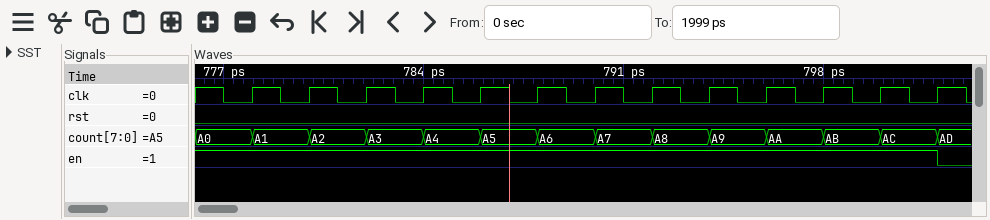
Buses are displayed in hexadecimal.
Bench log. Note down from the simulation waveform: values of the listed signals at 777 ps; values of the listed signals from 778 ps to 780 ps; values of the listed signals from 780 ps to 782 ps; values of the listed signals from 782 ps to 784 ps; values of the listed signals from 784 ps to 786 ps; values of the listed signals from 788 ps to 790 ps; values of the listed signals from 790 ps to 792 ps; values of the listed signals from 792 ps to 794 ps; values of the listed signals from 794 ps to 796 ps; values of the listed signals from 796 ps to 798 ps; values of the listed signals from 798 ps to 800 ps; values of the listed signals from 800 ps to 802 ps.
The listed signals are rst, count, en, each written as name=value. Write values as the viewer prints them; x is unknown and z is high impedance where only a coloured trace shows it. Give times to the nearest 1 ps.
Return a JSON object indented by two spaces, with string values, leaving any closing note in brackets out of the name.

{
  "values of the listed signals at 777 ps": "rst=0, count=A0, en=1",
  "values of the listed signals from 778 ps to 780 ps": "rst=0, count=A1, en=1",
  "values of the listed signals from 780 ps to 782 ps": "rst=0, count=A2, en=1",
  "values of the listed signals from 782 ps to 784 ps": "rst=0, count=A3, en=1",
  "values of the listed signals from 784 ps to 786 ps": "rst=0, count=A4, en=1",
  "values of the listed signals from 788 ps to 790 ps": "rst=0, count=A6, en=1",
  "values of the listed signals from 790 ps to 792 ps": "rst=0, count=A7, en=1",
  "values of the listed signals from 792 ps to 794 ps": "rst=0, count=A8, en=1",
  "values of the listed signals from 794 ps to 796 ps": "rst=0, count=A9, en=1",
  "values of the listed signals from 796 ps to 798 ps": "rst=0, count=AA, en=1",
  "values of the listed signals from 798 ps to 800 ps": "rst=0, count=AB, en=1",
  "values of the listed signals from 800 ps to 802 ps": "rst=0, count=AC, en=1"
}
